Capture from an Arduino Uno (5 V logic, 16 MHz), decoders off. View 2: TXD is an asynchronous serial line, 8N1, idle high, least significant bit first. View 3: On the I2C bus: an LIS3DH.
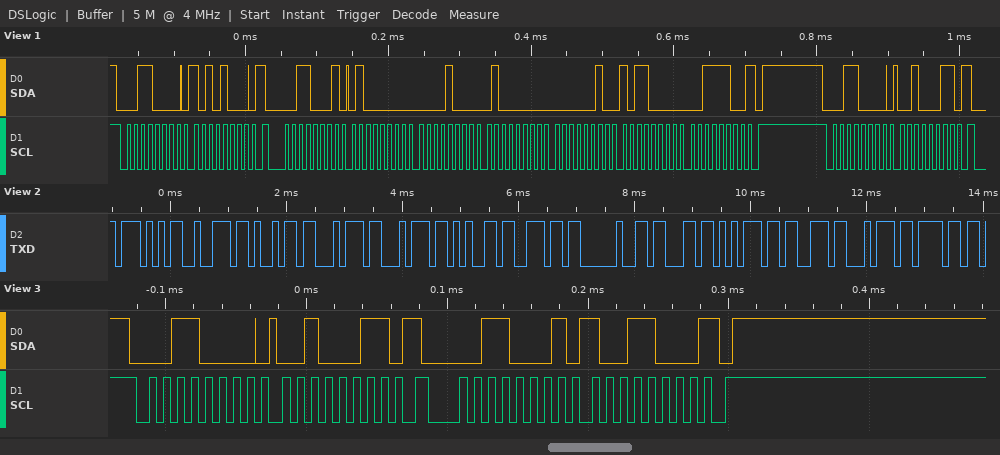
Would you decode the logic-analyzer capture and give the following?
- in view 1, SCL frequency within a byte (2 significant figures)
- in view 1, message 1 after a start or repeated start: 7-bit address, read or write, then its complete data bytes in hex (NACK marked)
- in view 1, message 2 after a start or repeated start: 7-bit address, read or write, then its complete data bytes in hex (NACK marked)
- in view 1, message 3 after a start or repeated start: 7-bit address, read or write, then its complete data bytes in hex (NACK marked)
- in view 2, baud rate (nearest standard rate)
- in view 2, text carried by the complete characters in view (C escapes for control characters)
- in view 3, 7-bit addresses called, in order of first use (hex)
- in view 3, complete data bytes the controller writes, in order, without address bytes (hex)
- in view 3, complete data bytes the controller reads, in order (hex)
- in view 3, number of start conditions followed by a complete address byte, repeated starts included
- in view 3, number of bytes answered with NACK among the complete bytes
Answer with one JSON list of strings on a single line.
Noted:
["100 kHz", "0x18 write: A8", "0x18 read: 40 08 40 02 B0 3C NACK", "0x18 write: 23", "9600 baud", "\"Written custo\"", "0x18", "23", "98", "2", "1"]
